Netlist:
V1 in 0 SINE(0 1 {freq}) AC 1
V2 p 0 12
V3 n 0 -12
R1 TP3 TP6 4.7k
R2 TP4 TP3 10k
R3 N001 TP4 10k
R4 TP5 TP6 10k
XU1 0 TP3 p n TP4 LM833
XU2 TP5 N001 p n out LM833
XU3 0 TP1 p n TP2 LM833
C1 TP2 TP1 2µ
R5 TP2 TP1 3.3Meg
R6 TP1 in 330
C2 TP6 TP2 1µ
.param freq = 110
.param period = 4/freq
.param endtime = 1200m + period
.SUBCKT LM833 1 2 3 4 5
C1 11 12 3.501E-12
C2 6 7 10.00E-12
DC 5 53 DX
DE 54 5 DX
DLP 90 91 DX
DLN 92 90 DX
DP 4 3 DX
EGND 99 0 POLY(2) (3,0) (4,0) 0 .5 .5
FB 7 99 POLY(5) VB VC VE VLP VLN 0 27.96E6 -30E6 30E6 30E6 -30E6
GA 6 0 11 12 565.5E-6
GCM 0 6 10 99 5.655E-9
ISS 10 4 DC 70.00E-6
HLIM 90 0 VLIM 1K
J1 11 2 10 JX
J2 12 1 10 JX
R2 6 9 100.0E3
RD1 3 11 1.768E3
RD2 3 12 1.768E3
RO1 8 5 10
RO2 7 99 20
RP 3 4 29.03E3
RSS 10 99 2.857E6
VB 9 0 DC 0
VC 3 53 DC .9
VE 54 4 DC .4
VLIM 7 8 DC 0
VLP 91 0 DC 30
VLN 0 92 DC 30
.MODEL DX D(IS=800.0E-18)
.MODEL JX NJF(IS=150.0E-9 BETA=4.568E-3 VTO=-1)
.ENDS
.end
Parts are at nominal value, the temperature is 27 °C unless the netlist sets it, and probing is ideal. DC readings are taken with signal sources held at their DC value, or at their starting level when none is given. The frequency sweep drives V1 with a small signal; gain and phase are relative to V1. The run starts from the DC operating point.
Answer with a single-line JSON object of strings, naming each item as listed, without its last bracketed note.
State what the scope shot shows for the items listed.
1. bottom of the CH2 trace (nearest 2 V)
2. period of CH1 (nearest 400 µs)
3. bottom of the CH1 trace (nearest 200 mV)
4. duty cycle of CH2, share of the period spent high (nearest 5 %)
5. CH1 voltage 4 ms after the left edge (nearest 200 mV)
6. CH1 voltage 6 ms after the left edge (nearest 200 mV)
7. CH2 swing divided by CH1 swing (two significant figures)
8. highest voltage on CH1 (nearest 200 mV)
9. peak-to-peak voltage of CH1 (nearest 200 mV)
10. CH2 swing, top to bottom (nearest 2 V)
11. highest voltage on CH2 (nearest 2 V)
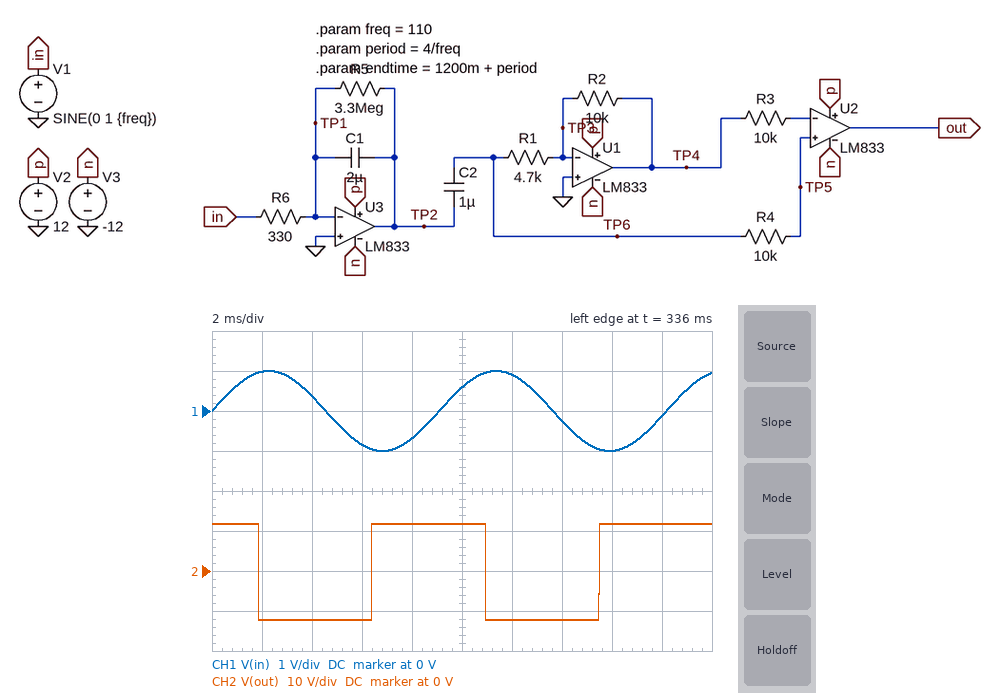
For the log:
{"bottom of the CH2 trace": "-12 V", "period of CH1": "9.2 ms", "bottom of the CH1 trace": "-1.0 V", "duty cycle of CH2, share of the period spent high": "50 %", "CH1 voltage 4 ms after the left edge": "400 mV", "CH1 voltage 6 ms after the left edge": "-800 mV", "CH2 swing divided by CH1 swing": "12", "highest voltage on CH1": "1.0 V", "peak-to-peak voltage of CH1": "2.0 V", "CH2 swing, top to bottom": "24 V", "highest voltage on CH2": "12 V"}
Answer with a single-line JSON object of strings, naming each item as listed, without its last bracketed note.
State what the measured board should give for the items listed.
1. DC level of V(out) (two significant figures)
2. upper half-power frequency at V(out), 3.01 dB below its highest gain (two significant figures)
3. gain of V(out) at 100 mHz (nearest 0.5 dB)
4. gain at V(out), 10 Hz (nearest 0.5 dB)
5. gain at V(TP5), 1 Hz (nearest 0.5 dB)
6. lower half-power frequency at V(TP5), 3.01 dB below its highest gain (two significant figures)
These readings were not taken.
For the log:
{"DC level of V(out)": "12 V", "upper half-power frequency at V(out), 3.01 dB below its highest gain": "34 Hz", "gain of V(out) at 100 mHz": "37.5 dB", "gain at V(out), 10 Hz": "37.5 dB", "gain at V(TP5), 1 Hz": "17.0 dB", "lower half-power frequency at V(TP5), 3.01 dB below its highest gain": "25 mHz"}
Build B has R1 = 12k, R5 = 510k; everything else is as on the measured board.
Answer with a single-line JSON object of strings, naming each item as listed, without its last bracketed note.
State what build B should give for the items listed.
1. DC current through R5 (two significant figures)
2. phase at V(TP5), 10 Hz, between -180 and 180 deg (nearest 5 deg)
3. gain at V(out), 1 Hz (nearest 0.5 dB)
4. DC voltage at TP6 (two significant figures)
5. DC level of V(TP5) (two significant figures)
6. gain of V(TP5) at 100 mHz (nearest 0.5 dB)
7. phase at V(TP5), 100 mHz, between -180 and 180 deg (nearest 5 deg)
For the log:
{"DC current through R5": "320 nA", "phase at V(TP5), 10 Hz, between -180 and 180 deg": "145 deg", "gain at V(out), 1 Hz": "39.0 dB", "DC voltage at TP6": "3.6 mV", "DC level of V(TP5)": "6.6 mV", "gain of V(TP5) at 100 mHz": "20.0 dB", "phase at V(TP5), 100 mHz, between -180 and 180 deg": "-125 deg"}
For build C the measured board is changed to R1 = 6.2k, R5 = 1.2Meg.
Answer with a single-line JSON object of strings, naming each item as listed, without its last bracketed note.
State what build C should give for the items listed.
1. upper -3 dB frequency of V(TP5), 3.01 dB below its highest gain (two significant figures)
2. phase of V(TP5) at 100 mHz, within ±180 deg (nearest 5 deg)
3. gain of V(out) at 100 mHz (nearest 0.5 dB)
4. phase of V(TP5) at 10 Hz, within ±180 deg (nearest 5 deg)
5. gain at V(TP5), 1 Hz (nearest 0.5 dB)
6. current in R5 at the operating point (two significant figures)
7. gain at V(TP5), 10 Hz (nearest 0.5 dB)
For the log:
{"upper -3 dB frequency of V(TP5), 3.01 dB below its highest gain": "26 Hz", "phase of V(TP5) at 100 mHz, within ±180 deg": "-145 deg", "gain of V(out) at 100 mHz": "36.5 dB", "phase of V(TP5) at 10 Hz, within ±180 deg": "160 deg", "gain at V(TP5), 1 Hz": "19.5 dB", "current in R5 at the operating point": "320 nA", "gain at V(TP5), 10 Hz": "19.0 dB"}
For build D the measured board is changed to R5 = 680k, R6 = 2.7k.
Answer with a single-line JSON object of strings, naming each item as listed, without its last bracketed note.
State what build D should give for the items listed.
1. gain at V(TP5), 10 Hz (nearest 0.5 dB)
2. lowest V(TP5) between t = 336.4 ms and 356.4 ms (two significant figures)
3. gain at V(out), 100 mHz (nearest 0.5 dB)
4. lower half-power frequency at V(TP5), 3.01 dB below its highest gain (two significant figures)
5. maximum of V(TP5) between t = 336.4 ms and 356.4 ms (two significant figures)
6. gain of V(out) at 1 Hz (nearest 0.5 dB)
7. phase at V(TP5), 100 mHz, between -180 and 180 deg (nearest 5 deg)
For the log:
{"gain at V(TP5), 10 Hz": "-1.5 dB", "lowest V(TP5) between t = 336.4 ms and 356.4 ms": "-250 mV", "gain at V(out), 100 mHz": "16.0 dB", "lower half-power frequency at V(TP5), 3.01 dB below its highest gain": "120 mHz", "maximum of V(TP5) between t = 336.4 ms and 356.4 ms": "260 mV", "gain of V(out) at 1 Hz": "19.5 dB", "phase at V(TP5), 100 mHz, between -180 and 180 deg": "-130 deg"}
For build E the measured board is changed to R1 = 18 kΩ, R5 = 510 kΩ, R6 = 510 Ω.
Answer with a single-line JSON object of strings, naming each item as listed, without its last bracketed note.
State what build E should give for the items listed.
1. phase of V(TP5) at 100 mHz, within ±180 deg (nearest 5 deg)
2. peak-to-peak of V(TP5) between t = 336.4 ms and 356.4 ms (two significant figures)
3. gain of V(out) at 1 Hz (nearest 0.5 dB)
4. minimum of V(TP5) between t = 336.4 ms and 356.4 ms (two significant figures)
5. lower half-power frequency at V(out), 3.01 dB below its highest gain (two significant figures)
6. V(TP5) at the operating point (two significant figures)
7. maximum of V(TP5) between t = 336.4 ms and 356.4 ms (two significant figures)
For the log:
{"phase of V(TP5) at 100 mHz, within ±180 deg": "-125 deg", "peak-to-peak of V(TP5) between t = 336.4 ms and 356.4 ms": "2.8 V", "gain of V(out) at 1 Hz": "35.5 dB", "minimum of V(TP5) between t = 336.4 ms and 356.4 ms": "-1.4 V", "lower half-power frequency at V(out), 3.01 dB below its highest gain": "150 mHz", "V(TP5) at the operating point": "8.4 mV", "maximum of V(TP5) between t = 336.4 ms and 356.4 ms": "1.4 V"}
